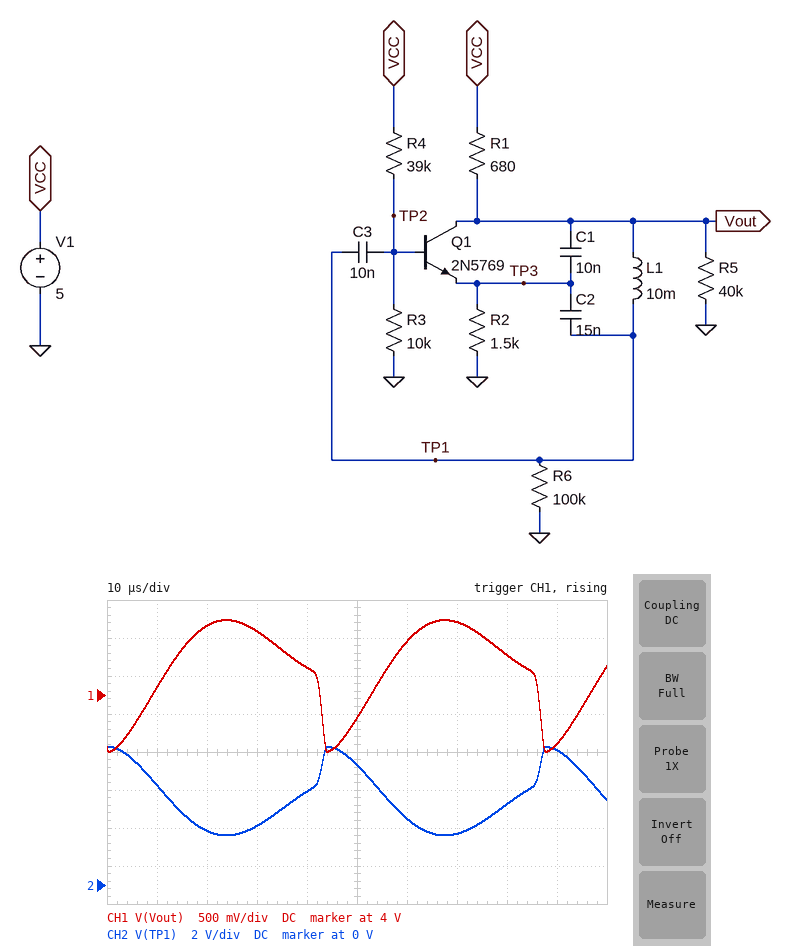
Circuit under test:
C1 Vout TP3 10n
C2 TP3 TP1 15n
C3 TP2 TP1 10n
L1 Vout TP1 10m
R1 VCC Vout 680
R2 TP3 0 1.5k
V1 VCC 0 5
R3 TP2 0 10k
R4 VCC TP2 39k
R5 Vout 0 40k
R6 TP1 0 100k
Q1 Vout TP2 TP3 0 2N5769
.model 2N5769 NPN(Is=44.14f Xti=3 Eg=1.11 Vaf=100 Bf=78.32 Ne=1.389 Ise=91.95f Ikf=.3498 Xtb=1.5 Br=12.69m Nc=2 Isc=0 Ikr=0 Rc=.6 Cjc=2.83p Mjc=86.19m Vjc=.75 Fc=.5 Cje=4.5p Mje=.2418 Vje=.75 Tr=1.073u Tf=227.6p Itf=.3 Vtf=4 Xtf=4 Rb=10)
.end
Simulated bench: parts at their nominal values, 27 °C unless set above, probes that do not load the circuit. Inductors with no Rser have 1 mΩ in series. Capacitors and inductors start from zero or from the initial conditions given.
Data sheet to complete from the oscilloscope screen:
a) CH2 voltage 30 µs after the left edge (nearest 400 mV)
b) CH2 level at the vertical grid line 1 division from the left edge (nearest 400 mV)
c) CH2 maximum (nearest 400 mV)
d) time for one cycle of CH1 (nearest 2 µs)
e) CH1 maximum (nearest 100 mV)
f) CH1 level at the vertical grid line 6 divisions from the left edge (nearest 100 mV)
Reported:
3.2 V
5.2 V
7.2 V
44 µs
5.0 V
4.7 V
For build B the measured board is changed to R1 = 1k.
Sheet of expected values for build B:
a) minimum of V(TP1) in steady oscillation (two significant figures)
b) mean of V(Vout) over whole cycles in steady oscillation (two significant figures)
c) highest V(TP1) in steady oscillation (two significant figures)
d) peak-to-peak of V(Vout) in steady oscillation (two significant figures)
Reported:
2.5 V
4.2 V
6.6 V
2.1 V
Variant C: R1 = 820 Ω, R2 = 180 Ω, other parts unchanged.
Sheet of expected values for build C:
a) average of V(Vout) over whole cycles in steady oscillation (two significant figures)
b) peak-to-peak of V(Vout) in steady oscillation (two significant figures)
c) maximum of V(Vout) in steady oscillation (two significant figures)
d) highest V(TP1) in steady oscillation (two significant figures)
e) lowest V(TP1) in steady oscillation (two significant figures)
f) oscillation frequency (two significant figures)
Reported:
3.5 V
3.8 V
4.8 V
4.5 V
2.8 V
29 kHz
